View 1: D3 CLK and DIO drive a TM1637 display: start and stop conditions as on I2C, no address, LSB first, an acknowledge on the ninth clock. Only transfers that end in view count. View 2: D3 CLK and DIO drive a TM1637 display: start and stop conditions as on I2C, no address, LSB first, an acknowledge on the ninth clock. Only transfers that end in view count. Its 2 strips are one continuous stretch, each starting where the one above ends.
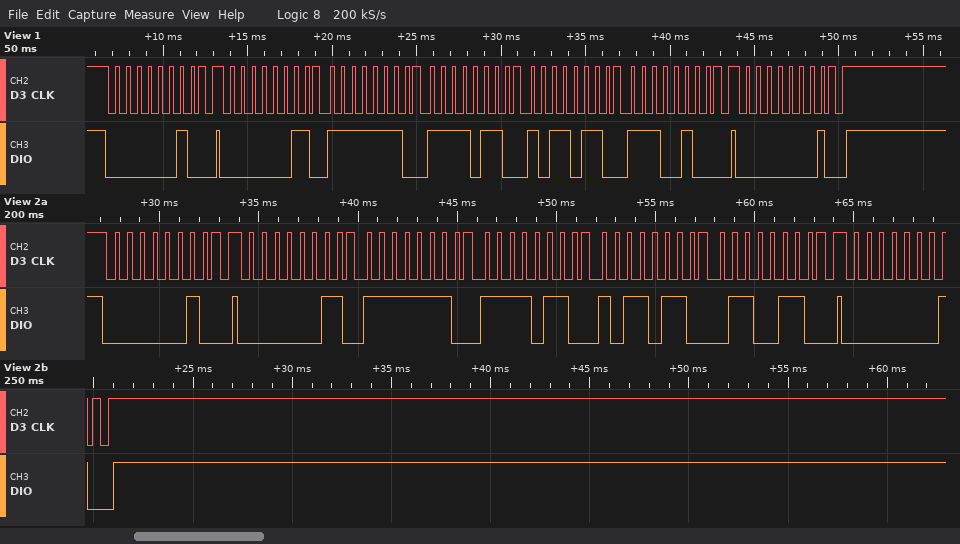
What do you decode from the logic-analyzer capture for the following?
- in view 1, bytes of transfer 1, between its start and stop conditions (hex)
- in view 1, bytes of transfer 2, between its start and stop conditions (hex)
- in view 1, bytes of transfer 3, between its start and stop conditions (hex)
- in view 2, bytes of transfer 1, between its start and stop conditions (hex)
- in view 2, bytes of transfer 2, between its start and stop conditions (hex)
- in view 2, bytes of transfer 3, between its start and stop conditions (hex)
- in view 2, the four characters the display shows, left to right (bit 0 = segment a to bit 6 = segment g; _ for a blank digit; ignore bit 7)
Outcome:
40
C0 7F 6F 6D 27
80
40
C0 7F 6F 6D 66
80
8954
